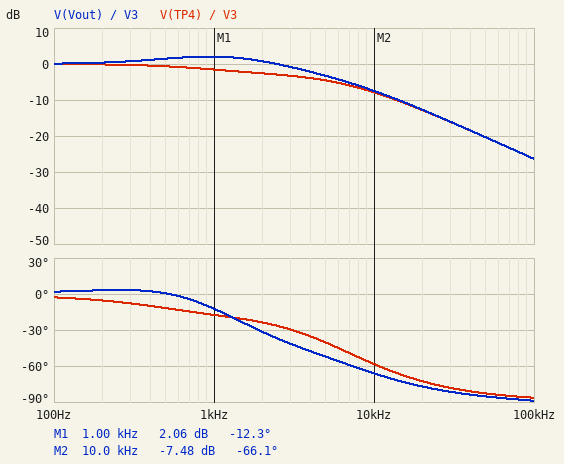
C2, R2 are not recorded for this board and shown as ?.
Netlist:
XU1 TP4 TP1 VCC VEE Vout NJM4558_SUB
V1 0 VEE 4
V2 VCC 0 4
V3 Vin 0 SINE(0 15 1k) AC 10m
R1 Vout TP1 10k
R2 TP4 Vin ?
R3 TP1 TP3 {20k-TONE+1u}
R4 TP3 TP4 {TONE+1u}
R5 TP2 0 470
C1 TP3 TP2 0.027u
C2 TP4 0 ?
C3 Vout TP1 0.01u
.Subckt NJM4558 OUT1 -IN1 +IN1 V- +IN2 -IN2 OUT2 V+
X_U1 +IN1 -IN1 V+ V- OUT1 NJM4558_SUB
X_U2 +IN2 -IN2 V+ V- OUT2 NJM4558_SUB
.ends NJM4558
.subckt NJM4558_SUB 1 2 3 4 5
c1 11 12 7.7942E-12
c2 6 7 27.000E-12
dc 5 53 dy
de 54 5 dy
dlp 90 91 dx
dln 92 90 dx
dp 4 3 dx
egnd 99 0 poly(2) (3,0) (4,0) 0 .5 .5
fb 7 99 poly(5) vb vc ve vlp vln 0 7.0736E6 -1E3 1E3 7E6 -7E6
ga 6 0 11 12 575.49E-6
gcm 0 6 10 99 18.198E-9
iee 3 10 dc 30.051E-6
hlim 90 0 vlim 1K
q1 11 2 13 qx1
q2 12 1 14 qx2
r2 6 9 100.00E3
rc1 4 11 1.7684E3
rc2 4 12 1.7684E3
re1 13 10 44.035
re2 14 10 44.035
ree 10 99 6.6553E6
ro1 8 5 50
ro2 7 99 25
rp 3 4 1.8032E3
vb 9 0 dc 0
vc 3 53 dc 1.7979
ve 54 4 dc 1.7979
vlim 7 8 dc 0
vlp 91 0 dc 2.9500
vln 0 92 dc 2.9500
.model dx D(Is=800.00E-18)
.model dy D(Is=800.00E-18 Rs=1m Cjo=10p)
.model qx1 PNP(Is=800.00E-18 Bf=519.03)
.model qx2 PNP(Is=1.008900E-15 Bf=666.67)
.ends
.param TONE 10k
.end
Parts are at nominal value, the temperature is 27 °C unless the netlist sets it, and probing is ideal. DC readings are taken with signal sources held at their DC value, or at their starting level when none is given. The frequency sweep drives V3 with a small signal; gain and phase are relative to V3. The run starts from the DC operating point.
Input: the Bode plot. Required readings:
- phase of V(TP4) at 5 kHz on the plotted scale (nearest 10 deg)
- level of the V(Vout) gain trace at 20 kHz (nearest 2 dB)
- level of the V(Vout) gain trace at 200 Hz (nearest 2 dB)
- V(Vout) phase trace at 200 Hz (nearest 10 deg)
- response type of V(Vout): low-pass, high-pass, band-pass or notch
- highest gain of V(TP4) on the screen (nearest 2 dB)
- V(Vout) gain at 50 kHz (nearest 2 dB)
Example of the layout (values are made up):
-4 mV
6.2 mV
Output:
-40 deg
-12 dB
0 dB
0 deg
low-pass
0 dB
-20 dB
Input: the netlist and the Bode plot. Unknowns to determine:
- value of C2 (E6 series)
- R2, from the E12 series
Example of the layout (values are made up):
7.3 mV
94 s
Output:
10 nF
3.3 kΩ
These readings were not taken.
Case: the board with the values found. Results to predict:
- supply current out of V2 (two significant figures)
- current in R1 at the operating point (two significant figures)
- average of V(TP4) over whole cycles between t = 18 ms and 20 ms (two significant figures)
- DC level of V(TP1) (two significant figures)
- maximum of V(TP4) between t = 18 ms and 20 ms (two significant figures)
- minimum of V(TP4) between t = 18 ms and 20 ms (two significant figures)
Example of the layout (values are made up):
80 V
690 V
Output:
4.5 mA
330 nA
1.3 V
-6.9 mV
12 V
-7.5 V
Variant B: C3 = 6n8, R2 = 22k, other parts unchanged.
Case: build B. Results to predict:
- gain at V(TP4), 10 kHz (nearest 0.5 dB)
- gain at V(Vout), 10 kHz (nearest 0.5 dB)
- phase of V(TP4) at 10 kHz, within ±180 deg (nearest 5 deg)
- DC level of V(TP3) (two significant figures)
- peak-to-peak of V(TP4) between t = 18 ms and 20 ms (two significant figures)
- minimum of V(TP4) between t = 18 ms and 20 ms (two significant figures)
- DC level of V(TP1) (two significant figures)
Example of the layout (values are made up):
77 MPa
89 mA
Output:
-23.0 dB
-22.5 dB
-80 deg
-9.1 mV
9.4 V
-4.6 V
-12 mV
